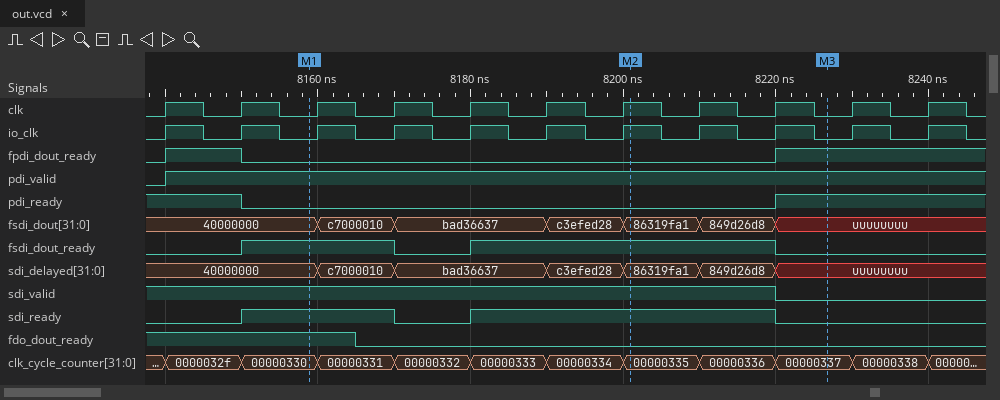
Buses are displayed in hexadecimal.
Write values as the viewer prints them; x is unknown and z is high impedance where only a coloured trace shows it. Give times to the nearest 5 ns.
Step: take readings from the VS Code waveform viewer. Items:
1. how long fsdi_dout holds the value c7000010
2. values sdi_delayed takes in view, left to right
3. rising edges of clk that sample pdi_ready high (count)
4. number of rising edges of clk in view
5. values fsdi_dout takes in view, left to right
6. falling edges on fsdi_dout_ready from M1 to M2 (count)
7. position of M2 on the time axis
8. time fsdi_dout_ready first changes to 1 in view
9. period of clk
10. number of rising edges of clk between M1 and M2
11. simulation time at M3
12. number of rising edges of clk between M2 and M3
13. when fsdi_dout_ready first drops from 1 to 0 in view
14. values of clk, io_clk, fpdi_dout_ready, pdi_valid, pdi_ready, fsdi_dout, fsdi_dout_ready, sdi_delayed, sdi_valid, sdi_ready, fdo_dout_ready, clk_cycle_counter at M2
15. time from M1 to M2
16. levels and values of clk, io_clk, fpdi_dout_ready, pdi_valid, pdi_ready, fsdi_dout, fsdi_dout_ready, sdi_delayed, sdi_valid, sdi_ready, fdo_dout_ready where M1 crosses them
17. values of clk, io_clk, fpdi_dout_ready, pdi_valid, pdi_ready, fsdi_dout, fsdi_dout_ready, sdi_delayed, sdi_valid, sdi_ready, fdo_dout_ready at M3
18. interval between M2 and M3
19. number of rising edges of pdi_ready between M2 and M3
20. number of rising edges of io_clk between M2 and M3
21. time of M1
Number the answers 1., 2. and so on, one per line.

1. 10 ns
2. 40000000, c7000010, bad36637, c3efed28, 86319fa1, 849d26d8, uuuuuuuu
3. 4
4. 11
5. 40000000, c7000010, bad36637, c3efed28, 86319fa1, 849d26d8, uuuuuuuu
6. 1
7. 8200 ns
8. 8150 ns
9. 10 ns
10. 5
11. 8225 ns
12. 2
13. 8170 ns
14. clk=1, io_clk=1, fpdi_dout_ready=0, pdi_valid=1, pdi_ready=0, fsdi_dout=86319fa1, fsdi_dout_ready=1, sdi_delayed=86319fa1, sdi_valid=1, sdi_ready=1, fdo_dout_ready=0, clk_cycle_counter=00000335
15. 40 ns
16. clk=0, io_clk=0, fpdi_dout_ready=0, pdi_valid=1, pdi_ready=0, fsdi_dout=40000000, fsdi_dout_ready=1, sdi_delayed=40000000, sdi_valid=1, sdi_ready=1, fdo_dout_ready=1
17. clk=0, io_clk=0, fpdi_dout_ready=1, pdi_valid=1, pdi_ready=1, fsdi_dout=uuuuuuuu, fsdi_dout_ready=0, sdi_delayed=uuuuuuuu, sdi_valid=0, sdi_ready=0, fdo_dout_ready=0
18. 25 ns
19. 1
20. 2
21. 8160 ns
